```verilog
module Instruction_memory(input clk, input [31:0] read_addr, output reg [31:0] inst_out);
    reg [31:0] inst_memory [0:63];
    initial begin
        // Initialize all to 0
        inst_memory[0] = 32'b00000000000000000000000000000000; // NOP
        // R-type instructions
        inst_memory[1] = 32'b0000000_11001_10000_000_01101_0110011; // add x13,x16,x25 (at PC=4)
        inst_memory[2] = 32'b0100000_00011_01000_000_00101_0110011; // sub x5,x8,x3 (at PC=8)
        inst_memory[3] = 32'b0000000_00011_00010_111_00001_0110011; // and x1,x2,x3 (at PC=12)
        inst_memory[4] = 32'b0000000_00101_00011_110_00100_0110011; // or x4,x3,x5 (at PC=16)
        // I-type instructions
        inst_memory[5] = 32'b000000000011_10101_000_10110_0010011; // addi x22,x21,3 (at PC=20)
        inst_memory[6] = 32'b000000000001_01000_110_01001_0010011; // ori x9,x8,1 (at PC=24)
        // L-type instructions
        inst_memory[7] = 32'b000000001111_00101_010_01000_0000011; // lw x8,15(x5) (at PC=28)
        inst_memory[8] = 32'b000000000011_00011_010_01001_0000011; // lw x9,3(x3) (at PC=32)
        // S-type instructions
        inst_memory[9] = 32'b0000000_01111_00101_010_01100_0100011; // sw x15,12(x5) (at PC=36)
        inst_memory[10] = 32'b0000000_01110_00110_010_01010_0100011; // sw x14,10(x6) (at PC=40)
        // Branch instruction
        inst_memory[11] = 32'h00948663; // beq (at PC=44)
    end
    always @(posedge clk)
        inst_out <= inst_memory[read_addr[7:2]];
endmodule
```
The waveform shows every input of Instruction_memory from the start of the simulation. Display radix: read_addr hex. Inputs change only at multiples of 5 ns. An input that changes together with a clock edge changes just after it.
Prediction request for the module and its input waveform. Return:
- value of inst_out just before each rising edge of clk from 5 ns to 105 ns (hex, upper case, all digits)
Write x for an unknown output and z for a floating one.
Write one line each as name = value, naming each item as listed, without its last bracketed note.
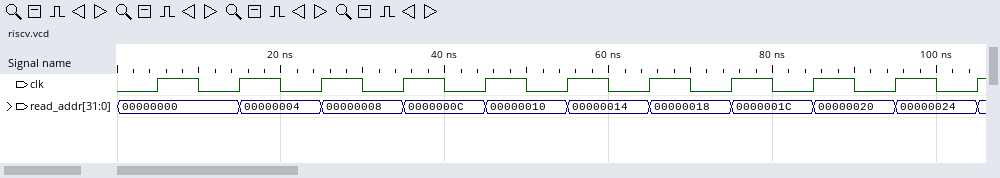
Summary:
value of inst_out just before each rising edge of clk from 5 ns to 105 ns = x, 00000000, 00000000, 019806B3, 403402B3, 003170B3, 0051E233, 003A8B13, 00146493, 00F2A403, 0031A483
